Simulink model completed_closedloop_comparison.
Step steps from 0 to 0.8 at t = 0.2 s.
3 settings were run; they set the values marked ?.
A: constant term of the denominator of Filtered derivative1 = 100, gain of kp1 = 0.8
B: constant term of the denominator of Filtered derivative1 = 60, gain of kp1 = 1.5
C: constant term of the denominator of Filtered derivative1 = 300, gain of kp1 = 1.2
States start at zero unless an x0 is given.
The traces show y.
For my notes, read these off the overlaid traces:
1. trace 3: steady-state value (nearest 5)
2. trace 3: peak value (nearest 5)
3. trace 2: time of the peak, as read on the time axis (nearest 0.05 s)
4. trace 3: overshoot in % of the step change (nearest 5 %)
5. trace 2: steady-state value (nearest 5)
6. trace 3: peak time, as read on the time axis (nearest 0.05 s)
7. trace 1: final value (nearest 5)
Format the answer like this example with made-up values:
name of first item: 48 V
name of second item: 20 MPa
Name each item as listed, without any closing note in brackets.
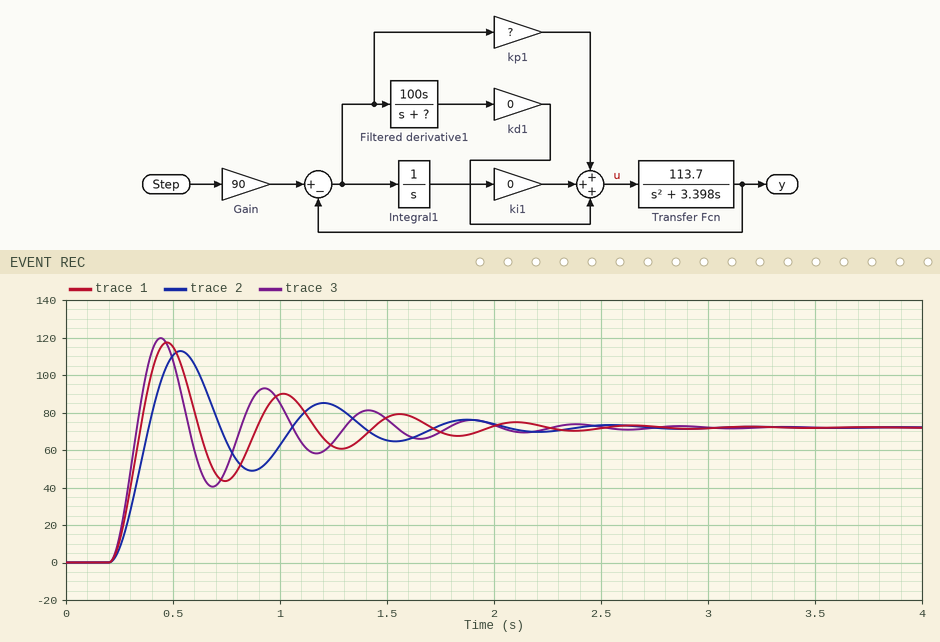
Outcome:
trace 3: steady-state value: 70
trace 3: peak value: 120
trace 2: time of the peak, as read on the time axis: 0.55 s
trace 3: overshoot in % of the step change: 65 %
trace 2: steady-state value: 70
trace 3: peak time, as read on the time axis: 0.45 s
trace 1: final value: 70
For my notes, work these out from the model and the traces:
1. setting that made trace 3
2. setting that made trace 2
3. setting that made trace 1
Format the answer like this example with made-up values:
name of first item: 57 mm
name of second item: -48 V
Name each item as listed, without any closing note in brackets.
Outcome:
setting that made trace 3: B
setting that made trace 2: A
setting that made trace 1: C
